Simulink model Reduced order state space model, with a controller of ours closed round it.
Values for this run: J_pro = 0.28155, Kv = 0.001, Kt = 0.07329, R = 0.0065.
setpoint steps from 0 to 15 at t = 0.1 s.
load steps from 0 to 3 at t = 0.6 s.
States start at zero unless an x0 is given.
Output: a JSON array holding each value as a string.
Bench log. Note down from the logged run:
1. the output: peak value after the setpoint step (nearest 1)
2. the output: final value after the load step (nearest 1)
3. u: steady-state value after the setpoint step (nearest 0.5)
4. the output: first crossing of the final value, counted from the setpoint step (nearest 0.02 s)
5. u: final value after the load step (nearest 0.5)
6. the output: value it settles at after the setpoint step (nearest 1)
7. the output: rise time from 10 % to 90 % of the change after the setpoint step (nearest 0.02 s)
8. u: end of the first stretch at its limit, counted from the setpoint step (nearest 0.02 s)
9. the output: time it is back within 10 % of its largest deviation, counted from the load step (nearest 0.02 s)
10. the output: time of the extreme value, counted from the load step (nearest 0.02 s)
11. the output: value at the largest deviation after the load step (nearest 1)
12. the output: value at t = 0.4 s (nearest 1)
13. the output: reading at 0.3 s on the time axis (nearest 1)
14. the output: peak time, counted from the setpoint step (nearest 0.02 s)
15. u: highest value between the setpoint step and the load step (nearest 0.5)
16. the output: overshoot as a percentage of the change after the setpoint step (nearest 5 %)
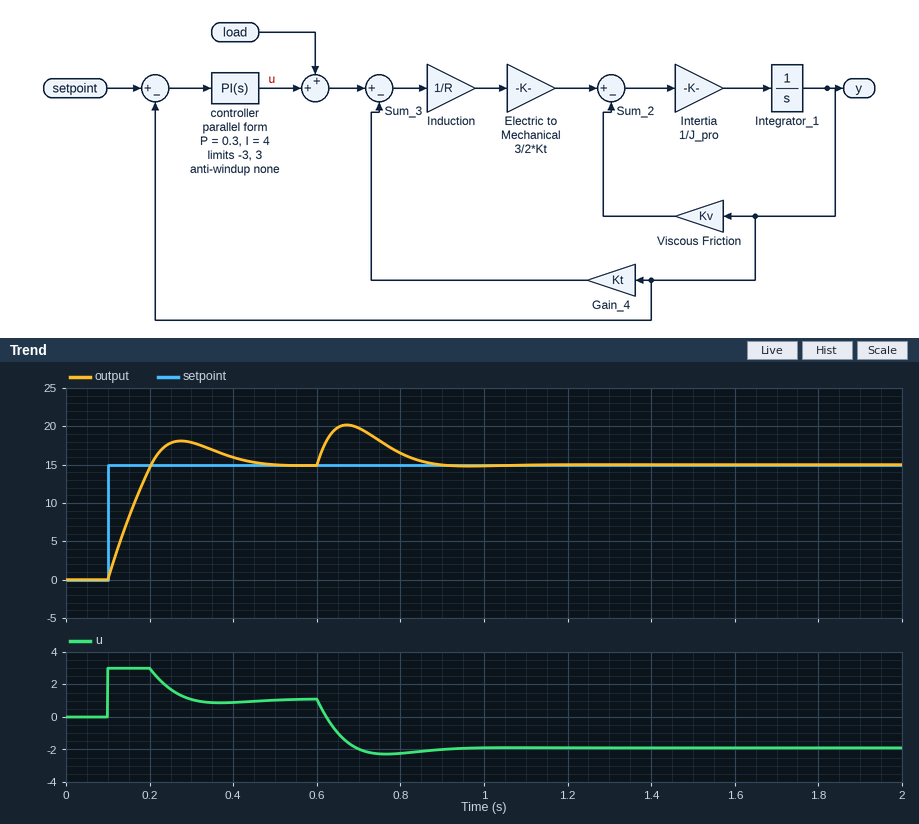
["18", "15", "1.0", "0.10 s", "-2.0", "15", "0.08 s", "0.10 s", "0.24 s", "0.08 s", "20", "16", "18", "0.18 s", "3.0", "20 %"]
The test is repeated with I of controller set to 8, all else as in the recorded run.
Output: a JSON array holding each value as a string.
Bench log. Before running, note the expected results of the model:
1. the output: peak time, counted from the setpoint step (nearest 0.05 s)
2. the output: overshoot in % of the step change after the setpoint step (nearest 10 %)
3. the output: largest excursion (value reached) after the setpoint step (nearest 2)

["0.20 s", "40 %", "22"]
